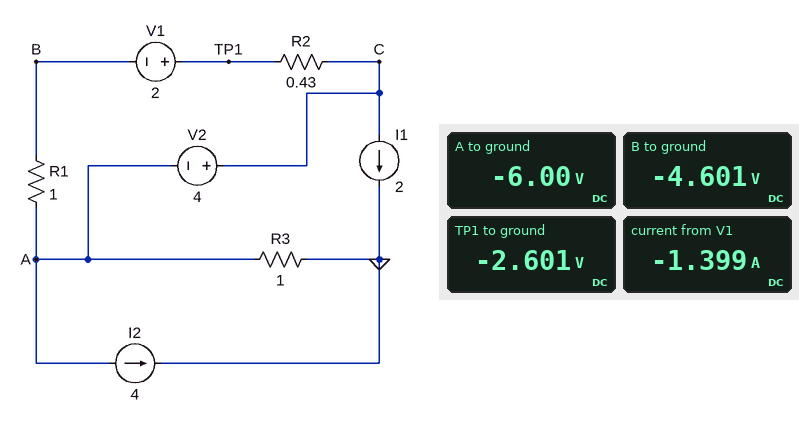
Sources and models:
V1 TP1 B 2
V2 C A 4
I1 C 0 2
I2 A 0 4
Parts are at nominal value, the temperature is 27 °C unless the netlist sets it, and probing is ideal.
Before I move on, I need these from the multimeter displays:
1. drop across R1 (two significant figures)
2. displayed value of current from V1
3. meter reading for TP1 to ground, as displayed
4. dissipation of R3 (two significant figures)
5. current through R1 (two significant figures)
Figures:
1.4 V
-1.399 A
-2.601 V
36 W
1.4 A
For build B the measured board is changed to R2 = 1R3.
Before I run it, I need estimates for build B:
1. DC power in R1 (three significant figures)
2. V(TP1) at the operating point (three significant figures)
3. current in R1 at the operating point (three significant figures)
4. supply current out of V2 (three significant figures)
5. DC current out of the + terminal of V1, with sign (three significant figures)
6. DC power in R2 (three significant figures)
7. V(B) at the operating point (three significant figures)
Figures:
756 mW
-3.13 V
870 mA
2.87 A
-870 mA
983 mW
-5.13 V
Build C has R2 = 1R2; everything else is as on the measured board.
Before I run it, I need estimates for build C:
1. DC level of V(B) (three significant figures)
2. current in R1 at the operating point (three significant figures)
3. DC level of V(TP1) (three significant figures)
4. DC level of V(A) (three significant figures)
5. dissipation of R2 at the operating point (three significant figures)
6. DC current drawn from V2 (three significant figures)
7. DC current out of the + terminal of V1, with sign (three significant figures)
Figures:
-5.09 V
909 mA
-3.09 V
-6.00 V
992 mW
2.91 A
-909 mA
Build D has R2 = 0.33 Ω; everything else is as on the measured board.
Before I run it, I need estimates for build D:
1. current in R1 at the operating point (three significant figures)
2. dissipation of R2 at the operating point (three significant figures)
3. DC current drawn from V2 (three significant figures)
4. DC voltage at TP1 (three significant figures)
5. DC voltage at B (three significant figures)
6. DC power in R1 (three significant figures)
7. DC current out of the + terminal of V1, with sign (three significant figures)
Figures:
1.50 A
746 mW
3.50 A
-2.50 V
-4.50 V
2.26 W
-1.50 A
